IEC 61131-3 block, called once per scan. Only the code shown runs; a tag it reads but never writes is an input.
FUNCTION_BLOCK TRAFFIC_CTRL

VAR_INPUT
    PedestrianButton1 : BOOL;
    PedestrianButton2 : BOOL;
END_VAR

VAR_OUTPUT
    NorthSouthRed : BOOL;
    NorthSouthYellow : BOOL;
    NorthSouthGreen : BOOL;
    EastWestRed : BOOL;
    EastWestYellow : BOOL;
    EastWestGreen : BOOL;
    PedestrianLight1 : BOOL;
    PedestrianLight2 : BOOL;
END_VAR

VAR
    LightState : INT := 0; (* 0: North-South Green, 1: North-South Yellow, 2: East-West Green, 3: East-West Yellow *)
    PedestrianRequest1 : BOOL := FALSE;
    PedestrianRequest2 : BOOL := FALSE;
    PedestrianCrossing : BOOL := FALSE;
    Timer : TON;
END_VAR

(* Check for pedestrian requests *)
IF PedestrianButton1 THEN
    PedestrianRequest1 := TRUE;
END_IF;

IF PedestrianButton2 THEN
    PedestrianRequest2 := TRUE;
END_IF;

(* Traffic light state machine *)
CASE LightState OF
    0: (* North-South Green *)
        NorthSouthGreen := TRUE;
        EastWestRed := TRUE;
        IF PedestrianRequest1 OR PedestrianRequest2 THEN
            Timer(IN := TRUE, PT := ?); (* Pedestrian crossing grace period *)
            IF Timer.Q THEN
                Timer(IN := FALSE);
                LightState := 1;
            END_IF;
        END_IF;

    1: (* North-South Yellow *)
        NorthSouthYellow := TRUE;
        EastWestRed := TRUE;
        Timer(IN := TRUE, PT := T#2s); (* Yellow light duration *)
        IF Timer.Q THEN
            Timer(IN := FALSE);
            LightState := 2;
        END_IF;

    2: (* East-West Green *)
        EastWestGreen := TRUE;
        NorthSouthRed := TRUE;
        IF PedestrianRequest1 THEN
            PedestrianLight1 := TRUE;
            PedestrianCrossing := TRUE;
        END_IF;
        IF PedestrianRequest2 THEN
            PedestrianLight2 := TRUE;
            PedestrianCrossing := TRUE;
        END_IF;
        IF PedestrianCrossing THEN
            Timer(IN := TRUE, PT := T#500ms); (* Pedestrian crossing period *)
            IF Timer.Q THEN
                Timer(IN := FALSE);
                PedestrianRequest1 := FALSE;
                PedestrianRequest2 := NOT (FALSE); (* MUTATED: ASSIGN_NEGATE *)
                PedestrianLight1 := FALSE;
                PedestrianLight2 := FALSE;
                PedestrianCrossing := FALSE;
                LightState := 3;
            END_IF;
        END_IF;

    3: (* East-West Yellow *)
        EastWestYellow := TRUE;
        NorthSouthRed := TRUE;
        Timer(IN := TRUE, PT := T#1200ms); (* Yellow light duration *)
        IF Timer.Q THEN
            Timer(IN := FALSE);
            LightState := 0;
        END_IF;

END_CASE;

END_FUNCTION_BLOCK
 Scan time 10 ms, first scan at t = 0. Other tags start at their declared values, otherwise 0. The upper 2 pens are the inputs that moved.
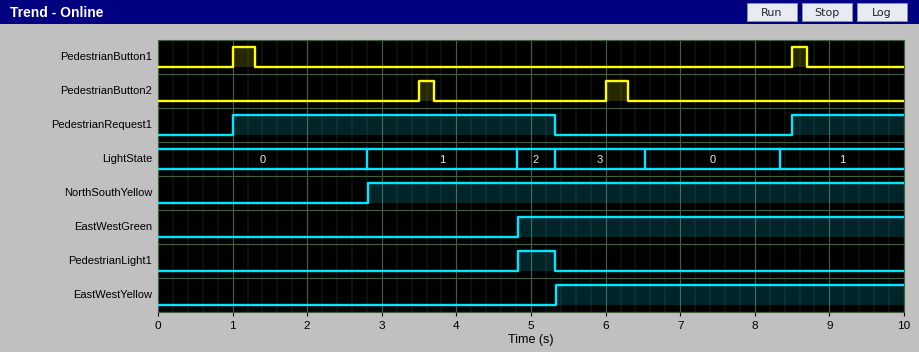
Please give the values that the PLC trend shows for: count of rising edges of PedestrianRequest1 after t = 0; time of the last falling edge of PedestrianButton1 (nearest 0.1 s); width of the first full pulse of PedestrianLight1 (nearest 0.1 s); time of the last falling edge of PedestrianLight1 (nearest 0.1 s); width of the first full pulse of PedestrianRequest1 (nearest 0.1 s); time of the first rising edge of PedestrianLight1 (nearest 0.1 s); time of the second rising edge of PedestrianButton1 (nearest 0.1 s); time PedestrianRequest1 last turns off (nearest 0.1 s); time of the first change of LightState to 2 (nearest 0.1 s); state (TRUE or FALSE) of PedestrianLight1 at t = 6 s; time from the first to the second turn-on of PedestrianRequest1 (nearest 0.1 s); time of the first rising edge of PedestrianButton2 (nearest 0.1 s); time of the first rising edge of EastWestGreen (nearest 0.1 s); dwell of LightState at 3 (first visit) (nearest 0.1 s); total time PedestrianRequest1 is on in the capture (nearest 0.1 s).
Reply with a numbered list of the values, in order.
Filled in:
1. 2
2. 8.7 s
3. 0.5 s
4. 5.3 s
5. 4.3 s
6. 4.8 s
7. 8.5 s
8. 5.3 s
9. 4.8 s
10. FALSE
11. 7.5 s
12. 3.5 s
13. 4.8 s
14. 1.2 s
15. 5.8 s
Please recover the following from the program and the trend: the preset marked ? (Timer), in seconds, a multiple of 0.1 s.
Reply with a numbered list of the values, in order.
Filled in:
1. 1.8 s
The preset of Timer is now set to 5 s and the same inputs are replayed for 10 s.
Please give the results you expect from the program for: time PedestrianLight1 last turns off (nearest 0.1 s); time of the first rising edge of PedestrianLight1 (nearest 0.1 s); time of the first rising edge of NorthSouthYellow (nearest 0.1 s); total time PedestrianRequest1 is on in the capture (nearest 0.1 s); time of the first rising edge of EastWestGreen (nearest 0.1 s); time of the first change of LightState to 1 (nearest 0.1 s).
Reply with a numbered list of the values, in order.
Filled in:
1. 8.5 s
2. 8.0 s
3. 6.0 s
4. 9.0 s
5. 8.0 s
6. 6.0 s
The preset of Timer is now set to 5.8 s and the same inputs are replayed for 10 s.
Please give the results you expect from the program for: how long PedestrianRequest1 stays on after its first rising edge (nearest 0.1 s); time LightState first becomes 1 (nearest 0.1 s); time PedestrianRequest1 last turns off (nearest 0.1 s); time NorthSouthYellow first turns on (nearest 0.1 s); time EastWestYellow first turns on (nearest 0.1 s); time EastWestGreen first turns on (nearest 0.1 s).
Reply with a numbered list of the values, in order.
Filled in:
1. 8.3 s
2. 6.8 s
3. 9.3 s
4. 6.8 s
5. 9.3 s
6. 8.8 s
